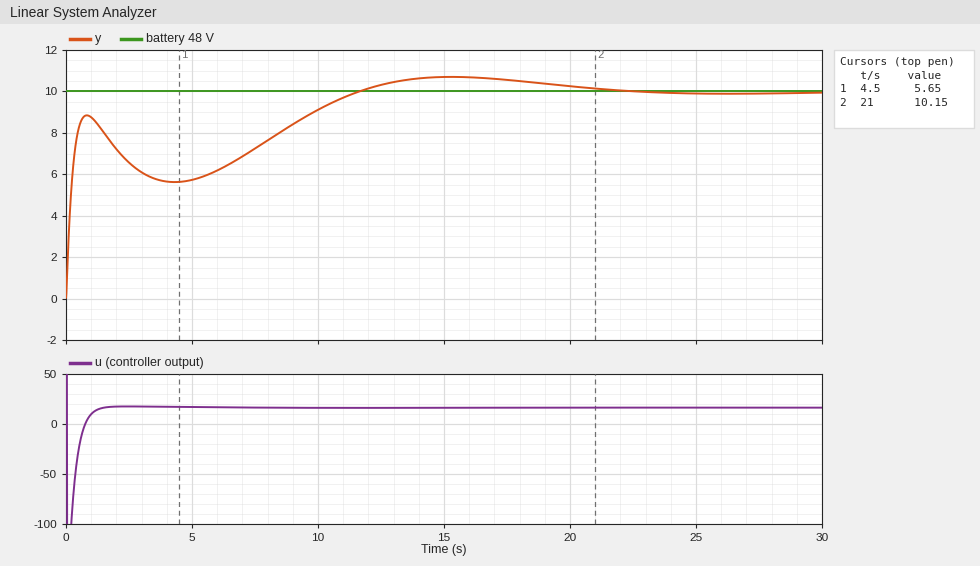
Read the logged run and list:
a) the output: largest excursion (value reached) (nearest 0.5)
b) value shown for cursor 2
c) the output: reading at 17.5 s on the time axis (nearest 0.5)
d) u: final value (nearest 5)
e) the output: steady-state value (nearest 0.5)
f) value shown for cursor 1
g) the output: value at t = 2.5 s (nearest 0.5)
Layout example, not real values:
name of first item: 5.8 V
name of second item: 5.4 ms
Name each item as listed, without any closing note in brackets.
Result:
the output: largest excursion (value reached): 10.5
value shown for cursor 2: 10.15
the output: reading at 17.5 s on the time axis: 10.5
u: final value: 15
the output: steady-state value: 10.0
value shown for cursor 1: 5.65
the output: value at t = 2.5 s: 6.5
